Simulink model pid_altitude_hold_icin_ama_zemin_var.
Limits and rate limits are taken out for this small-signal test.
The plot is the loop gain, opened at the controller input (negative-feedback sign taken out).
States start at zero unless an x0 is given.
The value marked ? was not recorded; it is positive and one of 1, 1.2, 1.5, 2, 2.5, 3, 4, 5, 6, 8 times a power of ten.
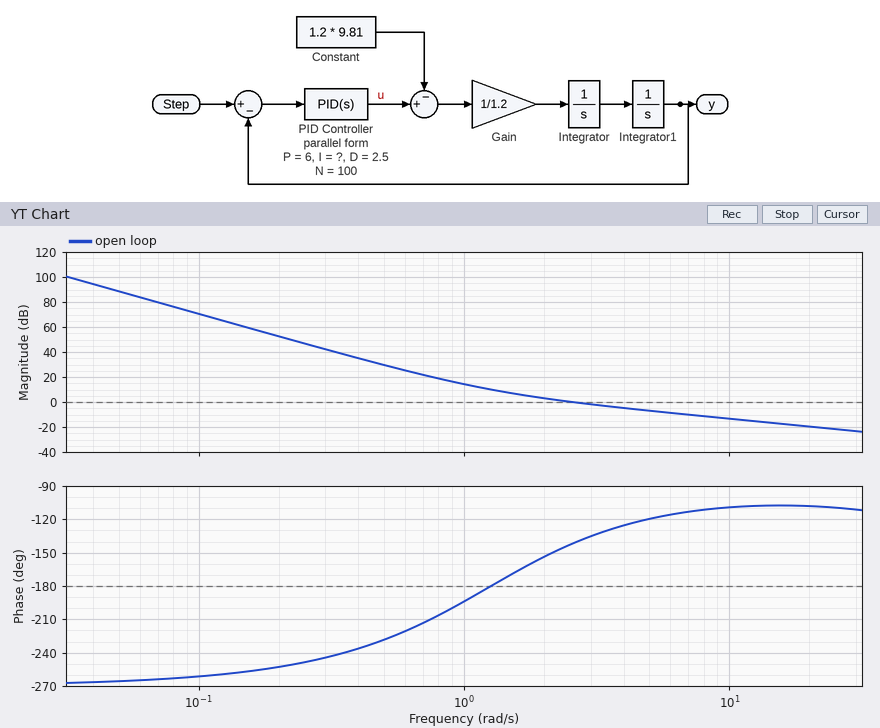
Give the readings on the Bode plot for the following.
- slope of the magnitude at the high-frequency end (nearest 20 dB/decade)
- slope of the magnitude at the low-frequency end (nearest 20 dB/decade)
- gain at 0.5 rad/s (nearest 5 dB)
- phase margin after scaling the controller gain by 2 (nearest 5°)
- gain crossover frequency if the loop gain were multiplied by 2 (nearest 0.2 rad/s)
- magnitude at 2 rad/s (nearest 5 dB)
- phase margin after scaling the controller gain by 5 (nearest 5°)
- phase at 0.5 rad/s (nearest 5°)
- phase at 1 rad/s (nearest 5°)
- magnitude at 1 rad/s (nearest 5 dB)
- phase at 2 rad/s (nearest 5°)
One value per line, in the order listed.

-20 dB/decade
-60 dB/decade
30 dB
60°
4.6 rad/s
5 dB
70°
-230°
-195°
15 dB
-155°
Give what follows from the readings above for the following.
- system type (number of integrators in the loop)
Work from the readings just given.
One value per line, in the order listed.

3
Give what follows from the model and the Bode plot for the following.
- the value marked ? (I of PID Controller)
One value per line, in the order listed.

4
